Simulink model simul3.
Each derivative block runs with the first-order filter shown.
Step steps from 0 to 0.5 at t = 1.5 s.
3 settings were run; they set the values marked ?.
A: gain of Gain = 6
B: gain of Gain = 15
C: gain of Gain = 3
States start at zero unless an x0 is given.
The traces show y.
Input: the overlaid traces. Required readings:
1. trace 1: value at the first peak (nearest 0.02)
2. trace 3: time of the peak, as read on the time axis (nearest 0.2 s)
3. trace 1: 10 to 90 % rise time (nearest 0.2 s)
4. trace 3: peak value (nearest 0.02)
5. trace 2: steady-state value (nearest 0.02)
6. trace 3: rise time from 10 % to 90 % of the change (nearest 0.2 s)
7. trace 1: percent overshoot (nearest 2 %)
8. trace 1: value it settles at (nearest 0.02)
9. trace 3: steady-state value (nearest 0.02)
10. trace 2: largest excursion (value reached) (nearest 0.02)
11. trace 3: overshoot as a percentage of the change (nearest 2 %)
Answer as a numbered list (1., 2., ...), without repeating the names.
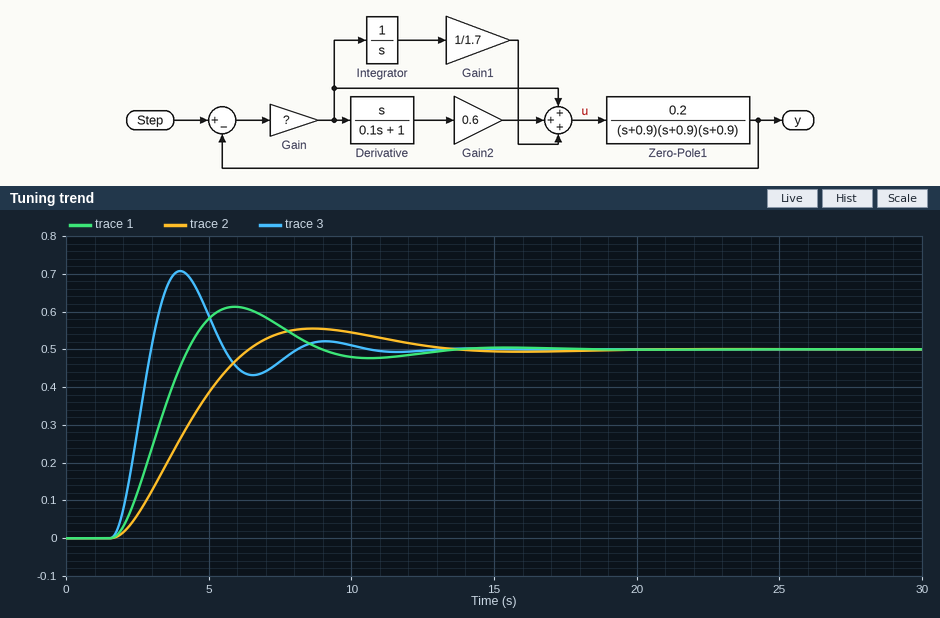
1. 0.62
2. 4.0 s
3. 1.8 s
4. 0.70
5. 0.50
6. 1.0 s
7. 22 %
8. 0.50
9. 0.50
10. 0.56
11. 42 %
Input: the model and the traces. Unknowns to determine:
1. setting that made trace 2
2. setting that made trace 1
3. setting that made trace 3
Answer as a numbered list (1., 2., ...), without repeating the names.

1. C
2. A
3. B
